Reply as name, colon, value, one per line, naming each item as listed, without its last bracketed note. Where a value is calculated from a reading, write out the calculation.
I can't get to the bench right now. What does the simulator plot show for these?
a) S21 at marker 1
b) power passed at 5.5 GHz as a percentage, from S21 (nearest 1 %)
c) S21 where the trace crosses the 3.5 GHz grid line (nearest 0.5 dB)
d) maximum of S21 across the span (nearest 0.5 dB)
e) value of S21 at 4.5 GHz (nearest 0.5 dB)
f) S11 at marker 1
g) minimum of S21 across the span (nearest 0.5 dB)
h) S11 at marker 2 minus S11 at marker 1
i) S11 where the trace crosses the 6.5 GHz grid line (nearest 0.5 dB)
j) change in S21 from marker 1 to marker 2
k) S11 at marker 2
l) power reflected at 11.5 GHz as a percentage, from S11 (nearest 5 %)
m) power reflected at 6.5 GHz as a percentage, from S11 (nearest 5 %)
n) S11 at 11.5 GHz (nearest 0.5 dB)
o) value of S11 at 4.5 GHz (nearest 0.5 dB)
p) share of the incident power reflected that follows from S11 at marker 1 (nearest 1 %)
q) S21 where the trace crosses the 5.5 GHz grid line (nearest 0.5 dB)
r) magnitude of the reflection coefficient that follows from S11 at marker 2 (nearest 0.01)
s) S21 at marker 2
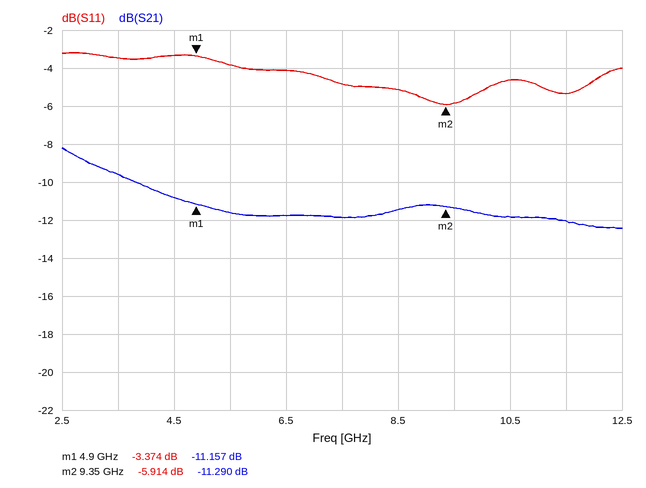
S21 at marker 1: -11.157 dB
power passed at 5.5 GHz as a percentage, from S21: 10^(-11.5/10) ≈ 7 %
S21 where the trace crosses the 3.5 GHz grid line: -9.5 dB
maximum of S21 across the span: -8.0 dB
value of S21 at 4.5 GHz: -11.0 dB
S11 at marker 1: -3.374 dB
minimum of S21 across the span: -12.5 dB
S11 at marker 2 minus S11 at marker 1: -5.914 − (-3.374) = -2.540 dB
S11 where the trace crosses the 6.5 GHz grid line: -4.0 dB
change in S21 from marker 1 to marker 2: -11.29 − (-11.157) = -0.133 dB
S11 at marker 2: -5.914 dB
power reflected at 11.5 GHz as a percentage, from S11: 10^(-5.5/10) ≈ 28.2 %, so 30 % to the nearest 5 %
power reflected at 6.5 GHz as a percentage, from S11: 10^(-4/10) ≈ 40 %
S11 at 11.5 GHz: -5.5 dB
value of S11 at 4.5 GHz: -3.5 dB
share of the incident power reflected that follows from S11 at marker 1: 10^(-3.374/10) ≈ 46 %
S21 where the trace crosses the 5.5 GHz grid line: -11.5 dB
magnitude of the reflection coefficient that follows from S11 at marker 2: 10^(-5.914/20) ≈ 0.51
S21 at marker 2: -11.290 dB
